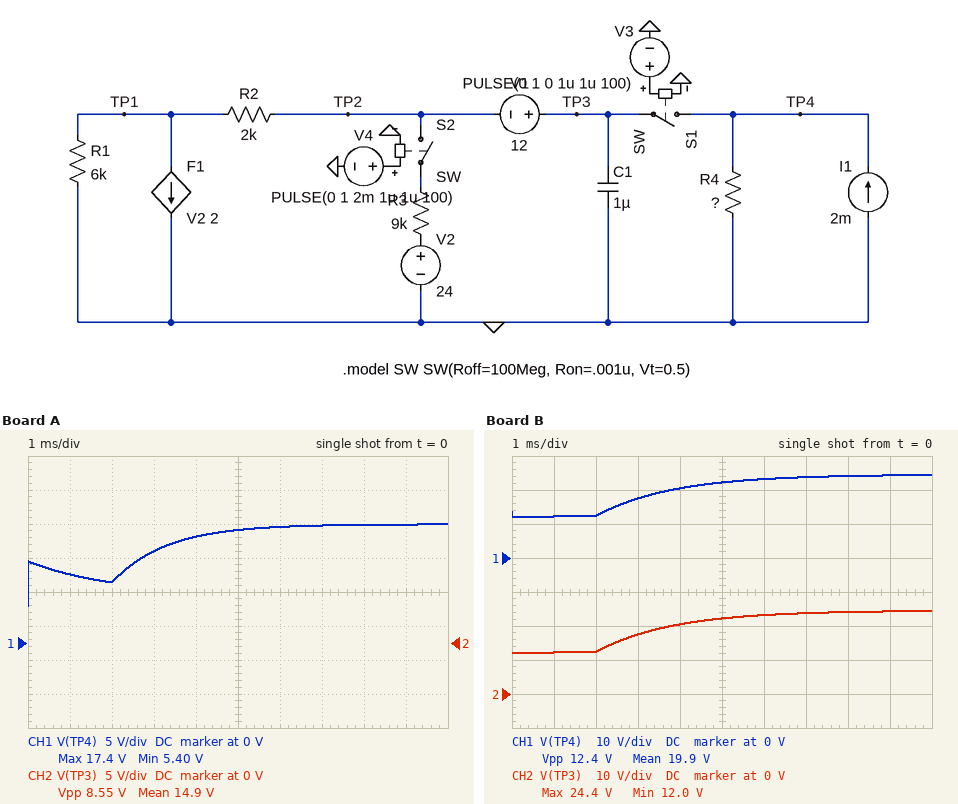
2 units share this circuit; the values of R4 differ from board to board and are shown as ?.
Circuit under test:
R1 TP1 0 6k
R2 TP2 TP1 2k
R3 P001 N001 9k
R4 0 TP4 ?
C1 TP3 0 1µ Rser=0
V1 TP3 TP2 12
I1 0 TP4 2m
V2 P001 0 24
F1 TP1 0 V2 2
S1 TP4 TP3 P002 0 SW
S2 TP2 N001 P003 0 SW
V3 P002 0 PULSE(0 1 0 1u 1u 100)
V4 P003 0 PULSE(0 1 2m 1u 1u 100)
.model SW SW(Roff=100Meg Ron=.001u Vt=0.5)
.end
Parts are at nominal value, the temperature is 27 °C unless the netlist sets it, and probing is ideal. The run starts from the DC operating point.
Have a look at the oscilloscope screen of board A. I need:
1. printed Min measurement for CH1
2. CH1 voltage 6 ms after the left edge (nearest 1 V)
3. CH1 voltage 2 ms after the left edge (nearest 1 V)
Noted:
5.40 V
17 V
9 V
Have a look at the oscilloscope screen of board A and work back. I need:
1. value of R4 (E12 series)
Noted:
2.7 kΩ
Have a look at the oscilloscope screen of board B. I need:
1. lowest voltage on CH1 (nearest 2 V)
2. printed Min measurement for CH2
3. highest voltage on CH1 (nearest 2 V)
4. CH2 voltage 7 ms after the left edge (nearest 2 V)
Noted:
12 V
12.0 V
24 V
24 V
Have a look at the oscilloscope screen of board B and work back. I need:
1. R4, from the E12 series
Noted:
6.8 kΩ
